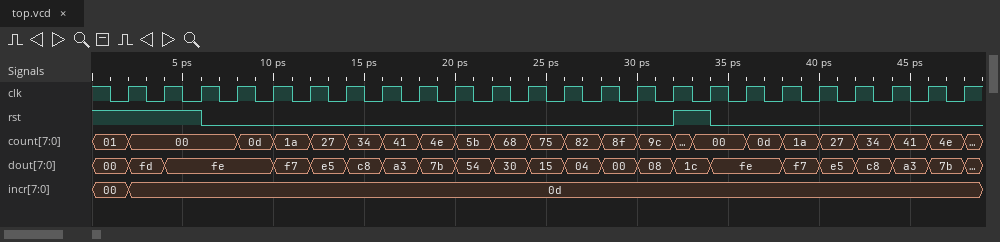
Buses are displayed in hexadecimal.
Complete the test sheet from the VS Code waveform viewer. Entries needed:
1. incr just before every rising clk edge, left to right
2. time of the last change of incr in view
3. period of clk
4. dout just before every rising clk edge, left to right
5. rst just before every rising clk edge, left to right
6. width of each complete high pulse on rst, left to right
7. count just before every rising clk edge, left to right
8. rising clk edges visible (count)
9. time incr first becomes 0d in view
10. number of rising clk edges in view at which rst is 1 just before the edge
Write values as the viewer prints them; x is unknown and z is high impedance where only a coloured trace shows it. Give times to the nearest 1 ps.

00, 0d, 0d, 0d, 0d, 0d, 0d, 0d, 0d, 0d, 0d, 0d, 0d, 0d, 0d, 0d, 0d, 0d, 0d, 0d, 0d, 0d, 0d, 0d
2 ps
2 ps
00, fd, fe, fe, fe, f7, e5, c8, a3, 7b, 54, 30, 15, 04, 00, 08, 1c, fe, fe, f7, e5, c8, a3, 7b
1 1 1 0 0 0 0 0 0 0 0 0 0 0 0 0 1 0 0 0 0 0 0 0
2 ps
01, 00, 00, 00, 0d, 1a, 27, 34, 41, 4e, 5b, 68, 75, 82, 8f, 9c, 00, 00, 0d, 1a, 27, 34, 41, 4e
24
2 ps
4
